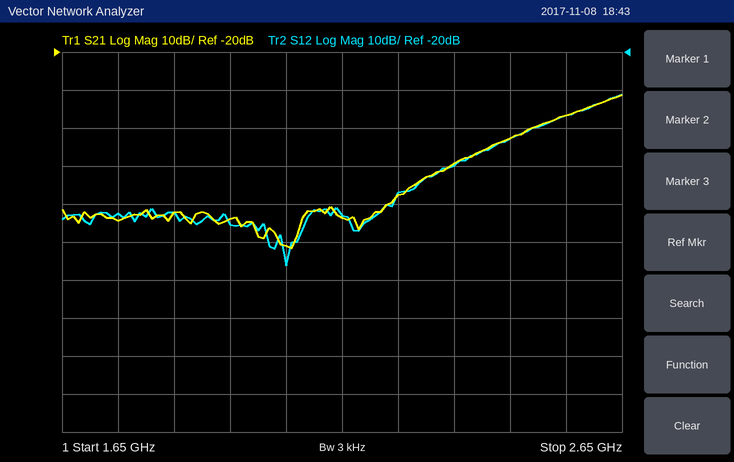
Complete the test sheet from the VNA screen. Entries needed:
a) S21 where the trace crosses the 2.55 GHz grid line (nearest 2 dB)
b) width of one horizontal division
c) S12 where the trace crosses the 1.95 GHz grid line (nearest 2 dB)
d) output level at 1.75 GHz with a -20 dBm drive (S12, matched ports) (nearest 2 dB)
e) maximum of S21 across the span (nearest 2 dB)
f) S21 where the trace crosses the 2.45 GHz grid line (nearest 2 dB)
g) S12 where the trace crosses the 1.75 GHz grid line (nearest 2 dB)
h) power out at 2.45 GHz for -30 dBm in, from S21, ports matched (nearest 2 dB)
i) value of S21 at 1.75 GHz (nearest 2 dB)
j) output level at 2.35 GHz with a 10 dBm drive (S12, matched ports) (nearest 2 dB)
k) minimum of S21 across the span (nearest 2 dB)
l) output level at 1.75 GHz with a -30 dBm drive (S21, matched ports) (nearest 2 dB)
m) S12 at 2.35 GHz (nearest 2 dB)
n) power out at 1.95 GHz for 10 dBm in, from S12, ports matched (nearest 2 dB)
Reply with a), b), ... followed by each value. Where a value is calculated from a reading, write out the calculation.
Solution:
a) -36 dB
b) 100 MHz
c) -66 dB
d) -20 dBm + (-62 dB) = -82 dBm
e) -32 dB
f) -42 dB
g) -62 dB
h) -30 dBm + (-42 dB) = -72 dBm
i) -64 dB
j) 10 dBm + (-50 dB) = -40 dBm
k) -72 dB
l) -30 dBm + (-64 dB) = -94 dBm
m) -50 dB
n) 10 dBm + (-66 dB) = -56 dBm
